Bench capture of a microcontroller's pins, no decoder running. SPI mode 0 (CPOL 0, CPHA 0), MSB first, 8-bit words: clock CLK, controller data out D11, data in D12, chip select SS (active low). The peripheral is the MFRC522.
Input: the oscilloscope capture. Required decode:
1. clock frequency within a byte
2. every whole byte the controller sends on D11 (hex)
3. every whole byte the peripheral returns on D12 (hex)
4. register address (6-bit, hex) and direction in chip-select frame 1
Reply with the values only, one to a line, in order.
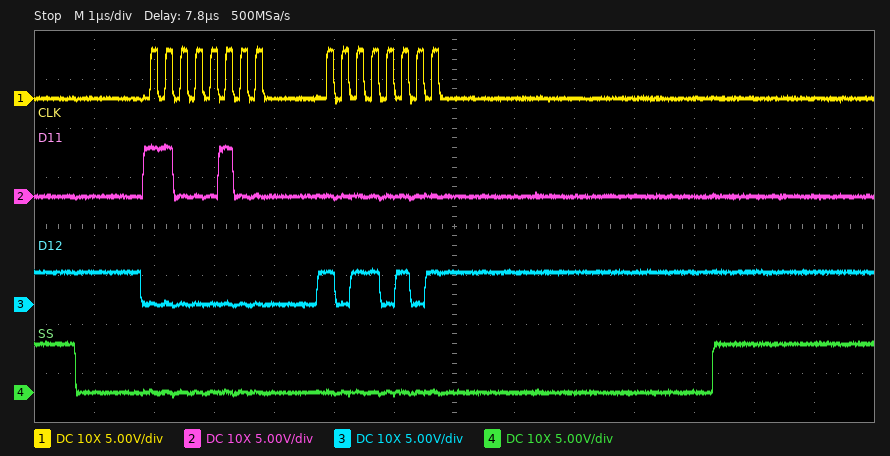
4 MHz
0xC4 0x00
0x00 0xB5
0x22 read
